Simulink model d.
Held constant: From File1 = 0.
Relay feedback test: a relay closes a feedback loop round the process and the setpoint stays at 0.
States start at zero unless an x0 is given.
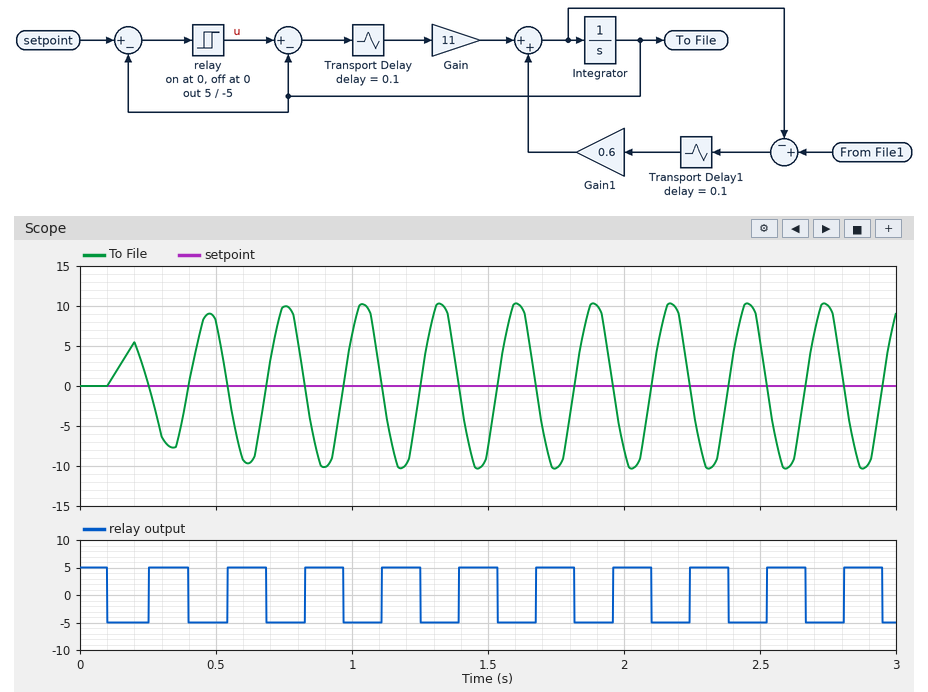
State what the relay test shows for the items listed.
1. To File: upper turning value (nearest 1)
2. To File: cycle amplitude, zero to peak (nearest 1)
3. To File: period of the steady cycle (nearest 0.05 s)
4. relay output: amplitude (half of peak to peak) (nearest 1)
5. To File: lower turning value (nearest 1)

10
10
0.30 s
5
-10
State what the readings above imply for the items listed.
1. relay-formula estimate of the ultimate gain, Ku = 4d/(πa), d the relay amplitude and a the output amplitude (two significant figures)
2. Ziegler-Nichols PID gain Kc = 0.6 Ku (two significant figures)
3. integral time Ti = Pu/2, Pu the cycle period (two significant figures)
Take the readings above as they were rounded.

0.64
0.38
0.15 s
